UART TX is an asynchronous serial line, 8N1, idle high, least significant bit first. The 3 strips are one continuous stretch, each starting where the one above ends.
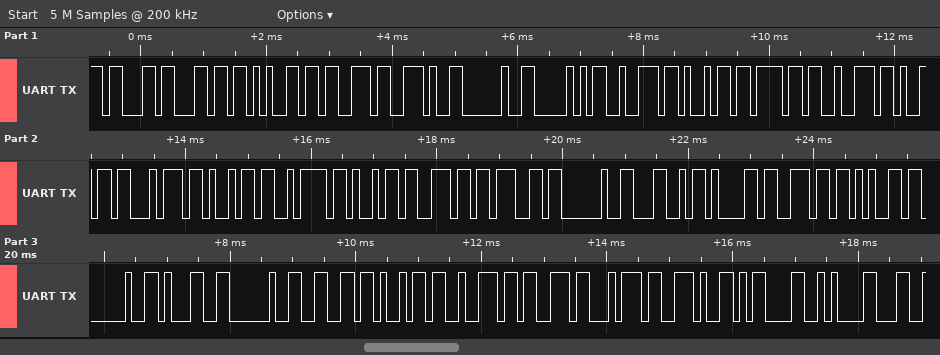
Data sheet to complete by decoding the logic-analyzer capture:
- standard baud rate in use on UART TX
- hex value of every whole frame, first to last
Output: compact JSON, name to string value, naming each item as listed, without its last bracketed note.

{"standard baud rate in use on UART TX": "9600 baud", "hex value of every whole frame, first to last": "63 6C 65 73 2E 20 50 72 69 6F 72 69 74 69 7A 69 6E 67 20 4C 61 6E 65 20 31 20 66 69 72 73 74 2E 0D 0A"}
